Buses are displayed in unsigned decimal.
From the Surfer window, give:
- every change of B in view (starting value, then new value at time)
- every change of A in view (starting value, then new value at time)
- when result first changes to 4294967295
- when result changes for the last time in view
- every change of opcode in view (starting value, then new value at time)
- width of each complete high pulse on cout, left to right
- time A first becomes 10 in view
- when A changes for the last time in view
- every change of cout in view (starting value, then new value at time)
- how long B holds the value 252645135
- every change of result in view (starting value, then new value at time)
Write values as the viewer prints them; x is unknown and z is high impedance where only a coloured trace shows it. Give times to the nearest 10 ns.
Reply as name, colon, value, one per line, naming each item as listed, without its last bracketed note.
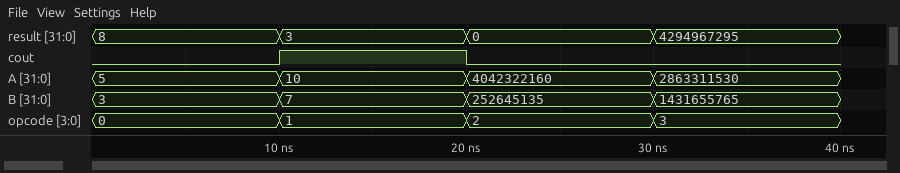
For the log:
every change of B in view: 3, 7 at 10 ns, 252645135 at 20 ns, 1431655765 at 30 ns
every change of A in view: 5, 10 at 10 ns, 4042322160 at 20 ns, 2863311530 at 30 ns
when result first changes to 4294967295: 30 ns
when result changes for the last time in view: 30 ns
every change of opcode in view: 0, 1 at 10 ns, 2 at 20 ns, 3 at 30 ns
width of each complete high pulse on cout, left to right: 10 ns
time A first becomes 10 in view: 10 ns
when A changes for the last time in view: 30 ns
every change of cout in view: 0, 1 at 10 ns, 0 at 20 ns
how long B holds the value 252645135: 10 ns
every change of result in view: 8, 3 at 10 ns, 0 at 20 ns, 4294967295 at 30 ns
